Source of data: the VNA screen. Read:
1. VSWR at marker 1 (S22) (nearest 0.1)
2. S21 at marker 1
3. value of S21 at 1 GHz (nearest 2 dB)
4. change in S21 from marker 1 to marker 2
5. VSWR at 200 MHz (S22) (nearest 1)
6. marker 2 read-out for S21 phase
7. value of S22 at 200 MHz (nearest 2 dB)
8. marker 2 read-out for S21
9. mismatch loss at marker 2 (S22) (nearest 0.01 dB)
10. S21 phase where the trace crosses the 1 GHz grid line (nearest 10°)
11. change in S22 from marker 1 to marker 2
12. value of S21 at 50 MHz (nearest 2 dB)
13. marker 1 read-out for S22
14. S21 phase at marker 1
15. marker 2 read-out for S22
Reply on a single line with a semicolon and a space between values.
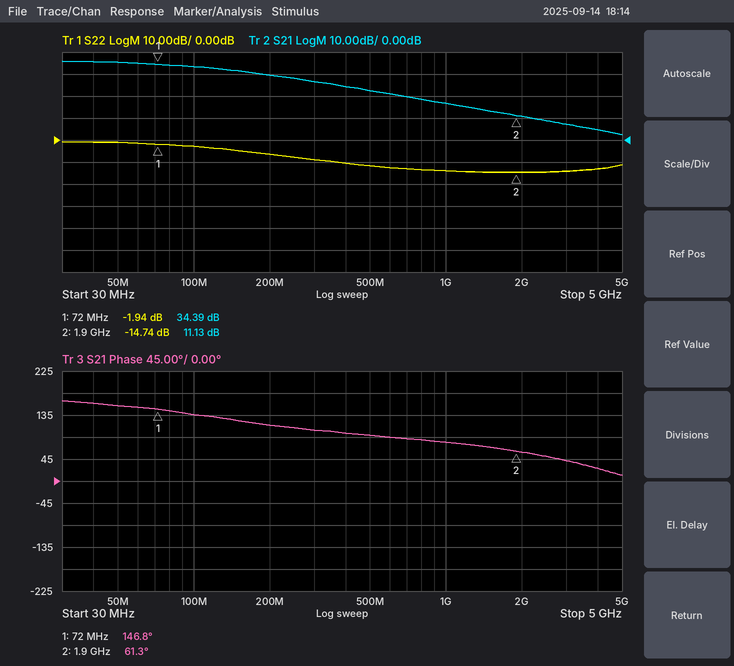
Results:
9.0; 34.39 dB; 16 dB; -23.26 dB; 3; 61.3°; -6 dB; 11.13 dB; 0.15 dB; 80°; -12.80 dB; 36 dB; -1.94 dB; 146.8°; -14.74 dB
